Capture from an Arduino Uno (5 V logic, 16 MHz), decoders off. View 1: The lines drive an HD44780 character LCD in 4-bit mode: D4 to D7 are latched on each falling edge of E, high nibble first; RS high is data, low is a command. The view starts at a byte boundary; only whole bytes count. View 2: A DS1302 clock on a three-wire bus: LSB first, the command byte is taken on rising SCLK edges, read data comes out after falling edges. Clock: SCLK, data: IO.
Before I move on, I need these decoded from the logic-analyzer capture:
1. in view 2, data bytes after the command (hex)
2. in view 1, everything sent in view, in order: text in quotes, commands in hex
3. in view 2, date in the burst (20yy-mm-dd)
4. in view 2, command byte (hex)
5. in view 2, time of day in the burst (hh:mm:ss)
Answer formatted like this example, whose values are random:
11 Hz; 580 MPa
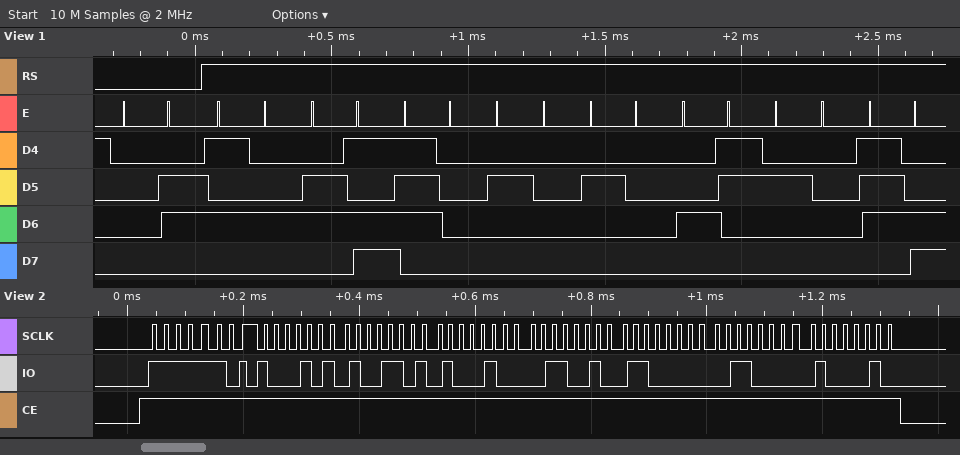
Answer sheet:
51 59 11 26 03 06 21; 0x06 "Tmp  C |"; 2021-03-26; 0xBF; 11:59:51
